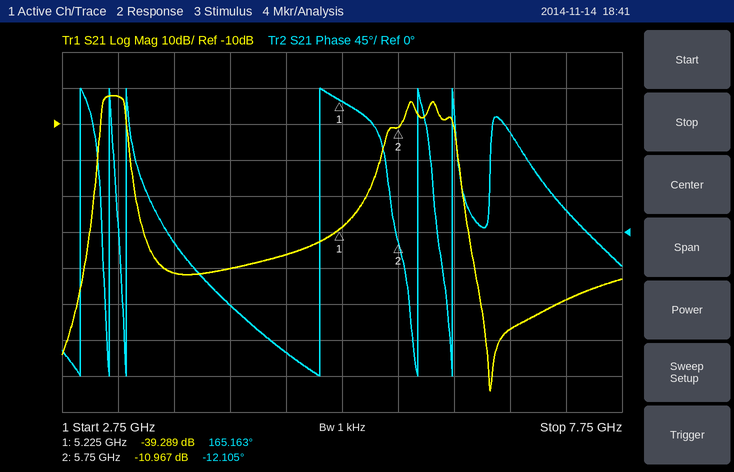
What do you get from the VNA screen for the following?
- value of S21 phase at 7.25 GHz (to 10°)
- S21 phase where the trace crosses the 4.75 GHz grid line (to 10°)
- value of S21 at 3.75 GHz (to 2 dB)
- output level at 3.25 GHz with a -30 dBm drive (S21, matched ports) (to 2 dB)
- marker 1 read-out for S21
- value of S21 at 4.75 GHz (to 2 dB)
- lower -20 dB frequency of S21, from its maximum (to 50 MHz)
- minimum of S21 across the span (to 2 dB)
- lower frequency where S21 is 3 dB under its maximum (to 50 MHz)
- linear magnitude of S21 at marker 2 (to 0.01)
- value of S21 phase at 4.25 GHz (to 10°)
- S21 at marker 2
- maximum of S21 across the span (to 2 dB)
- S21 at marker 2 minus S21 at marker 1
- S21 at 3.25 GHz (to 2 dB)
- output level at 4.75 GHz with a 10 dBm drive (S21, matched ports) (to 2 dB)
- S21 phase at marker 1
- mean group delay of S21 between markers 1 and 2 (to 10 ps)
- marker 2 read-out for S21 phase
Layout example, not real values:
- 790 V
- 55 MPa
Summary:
- 30°
- -150°
- -52 dB
- -32 dBm
- -39.289 dB
- -46 dB
- 3.05 GHz
- -84 dB
- 3.10 GHz
- 0.28
- -90°
- -10.967 dB
- -2 dB
- 28.322 dB
- -2 dB
- -36 dBm
- 165.163°
- 940 ps
- -12.105°
